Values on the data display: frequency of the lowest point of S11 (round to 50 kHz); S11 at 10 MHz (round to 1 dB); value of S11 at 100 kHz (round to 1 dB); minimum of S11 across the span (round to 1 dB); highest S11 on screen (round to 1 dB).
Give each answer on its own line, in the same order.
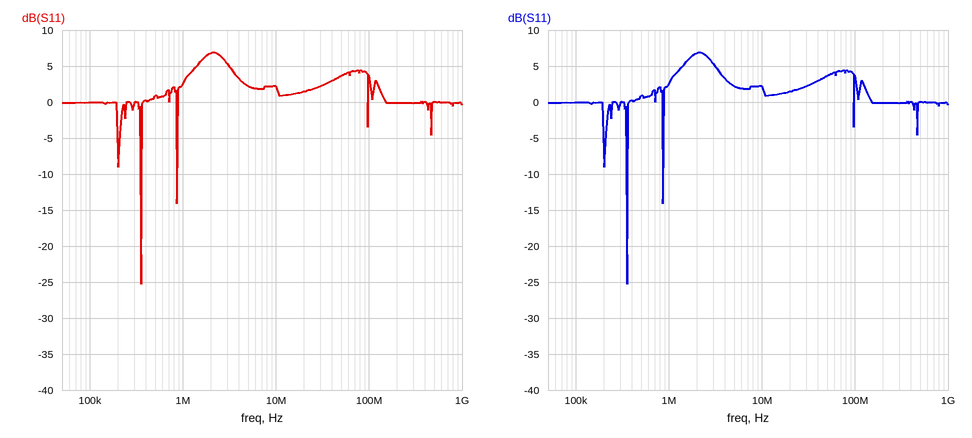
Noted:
350 kHz
2 dB
0 dB
-25 dB
7 dB
